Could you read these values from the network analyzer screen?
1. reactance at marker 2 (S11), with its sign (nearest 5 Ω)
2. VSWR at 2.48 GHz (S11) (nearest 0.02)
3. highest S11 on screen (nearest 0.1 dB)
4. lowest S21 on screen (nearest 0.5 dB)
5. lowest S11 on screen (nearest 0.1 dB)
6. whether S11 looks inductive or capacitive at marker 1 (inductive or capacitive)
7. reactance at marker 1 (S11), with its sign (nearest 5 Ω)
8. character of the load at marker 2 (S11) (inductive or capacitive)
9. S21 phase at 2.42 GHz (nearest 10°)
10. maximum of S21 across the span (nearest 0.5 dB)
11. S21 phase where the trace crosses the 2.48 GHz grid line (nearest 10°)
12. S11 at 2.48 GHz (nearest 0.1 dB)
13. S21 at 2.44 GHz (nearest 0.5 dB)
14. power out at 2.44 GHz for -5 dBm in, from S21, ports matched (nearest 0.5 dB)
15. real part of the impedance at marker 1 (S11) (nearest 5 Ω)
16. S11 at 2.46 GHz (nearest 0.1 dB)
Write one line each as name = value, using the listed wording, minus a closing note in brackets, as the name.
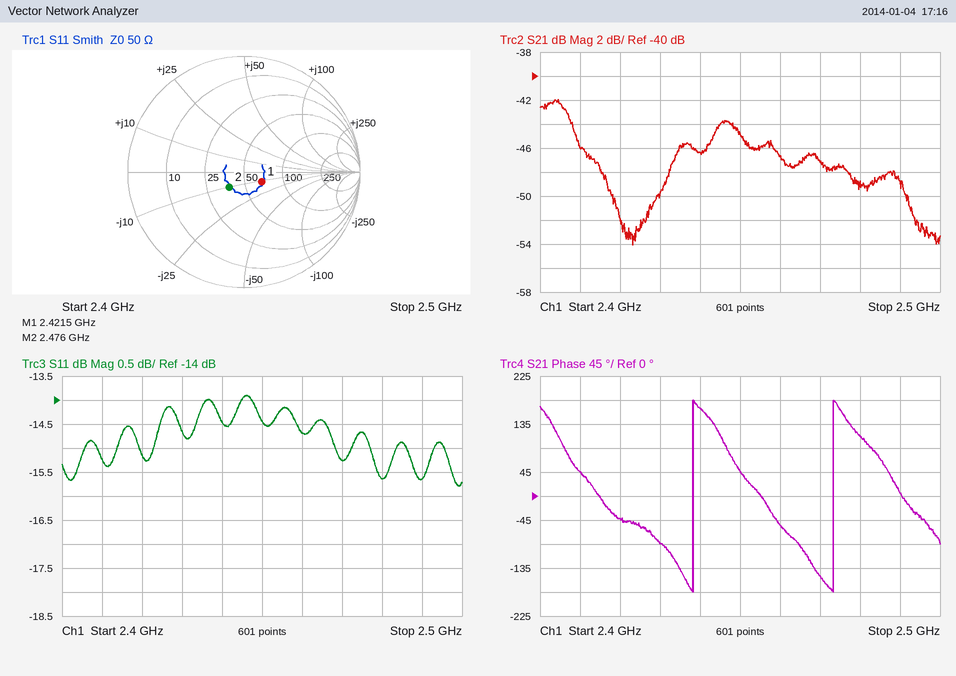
reactance at marker 2 (S11), with its sign = -10 Ω
VSWR at 2.48 GHz (S11) = 1.40
highest S11 on screen = -13.9 dB
lowest S21 on screen = -54.0 dB
lowest S11 on screen = -15.8 dB
whether S11 looks inductive or capacitive at marker 1 = capacitive
reactance at marker 1 (S11), with its sign = -10 Ω
character of the load at marker 2 (S11) = capacitive
S21 phase at 2.42 GHz = -40°
maximum of S21 across the span = -42.0 dB
S21 phase where the trace crosses the 2.48 GHz grid line = 110°
S11 at 2.48 GHz = -15.6 dB
S21 at 2.44 GHz = -46.5 dB
power out at 2.44 GHz for -5 dBm in, from S21, ports matched = -51.5 dBm
real part of the impedance at marker 1 (S11) = 65 Ω
S11 at 2.46 GHz = -14.7 dB
